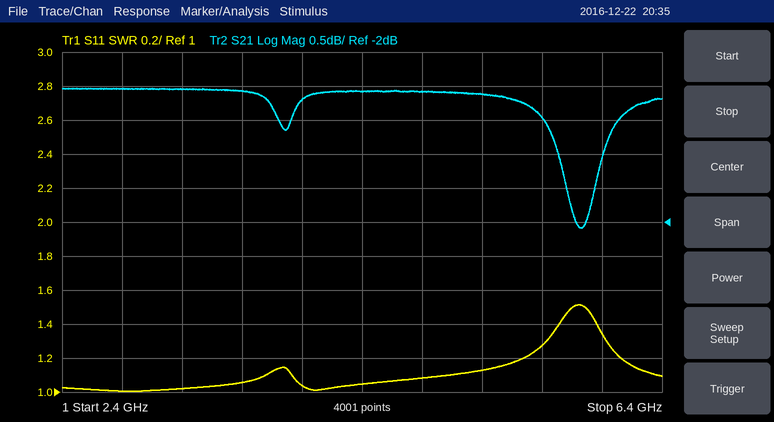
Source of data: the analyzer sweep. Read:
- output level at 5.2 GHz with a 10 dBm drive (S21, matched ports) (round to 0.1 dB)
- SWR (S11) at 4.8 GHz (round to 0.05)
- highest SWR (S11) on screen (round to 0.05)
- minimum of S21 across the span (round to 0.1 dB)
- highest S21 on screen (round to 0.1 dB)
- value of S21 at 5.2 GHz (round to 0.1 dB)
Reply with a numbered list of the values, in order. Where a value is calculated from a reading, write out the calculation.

1. 10 dBm + (-0.1 dB) = 9.9 dBm
2. 1.10
3. 1.50
4. -2.1 dB
5. 0.0 dB
6. -0.1 dB
